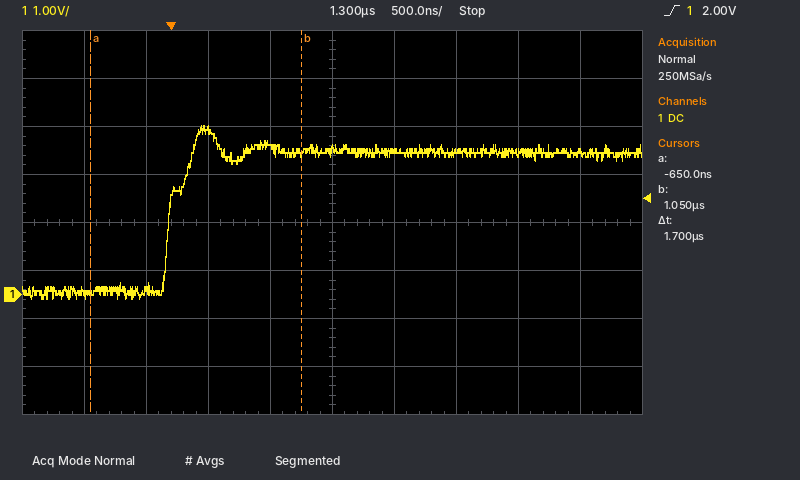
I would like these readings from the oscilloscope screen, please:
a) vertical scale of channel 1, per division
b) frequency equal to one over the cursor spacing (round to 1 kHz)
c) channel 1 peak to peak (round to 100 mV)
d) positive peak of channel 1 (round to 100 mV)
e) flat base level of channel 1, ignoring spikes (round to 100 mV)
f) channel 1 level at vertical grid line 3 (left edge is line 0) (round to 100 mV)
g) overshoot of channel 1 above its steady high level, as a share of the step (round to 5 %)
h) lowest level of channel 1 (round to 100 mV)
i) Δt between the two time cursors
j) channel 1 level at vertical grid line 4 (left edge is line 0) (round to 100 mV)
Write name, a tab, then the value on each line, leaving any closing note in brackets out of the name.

vertical scale of channel 1, per division	1 V
frequency equal to one over the cursor spacing	588 kHz
channel 1 peak to peak	3.6 V
positive peak of channel 1	3.5 V
flat base level of channel 1, ignoring spikes	100 mV
channel 1 level at vertical grid line 3 (left edge is line 0)	3.4 V
overshoot of channel 1 above its steady high level, as a share of the step	20 %
lowest level of channel 1	-100 mV
Δt between the two time cursors	1.7 µs
channel 1 level at vertical grid line 4 (left edge is line 0)	3.1 V
